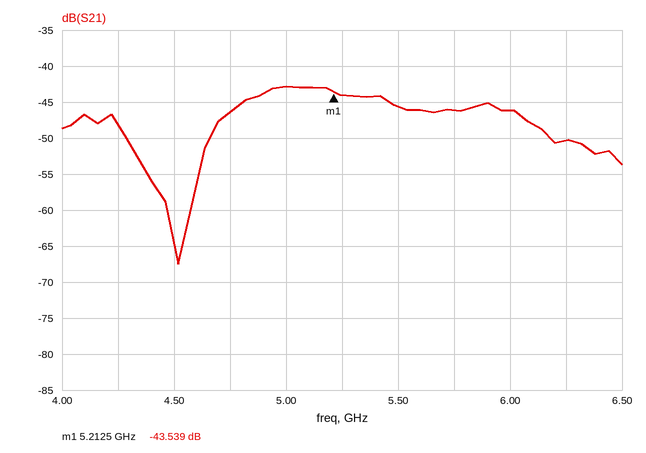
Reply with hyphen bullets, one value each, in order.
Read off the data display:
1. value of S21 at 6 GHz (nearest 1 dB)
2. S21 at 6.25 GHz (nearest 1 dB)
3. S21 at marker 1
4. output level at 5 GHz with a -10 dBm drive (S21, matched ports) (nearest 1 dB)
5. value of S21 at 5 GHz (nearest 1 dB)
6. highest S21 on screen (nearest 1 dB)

- -46 dB
- -50 dB
- -43.539 dB
- -53 dBm
- -43 dB
- -43 dB
